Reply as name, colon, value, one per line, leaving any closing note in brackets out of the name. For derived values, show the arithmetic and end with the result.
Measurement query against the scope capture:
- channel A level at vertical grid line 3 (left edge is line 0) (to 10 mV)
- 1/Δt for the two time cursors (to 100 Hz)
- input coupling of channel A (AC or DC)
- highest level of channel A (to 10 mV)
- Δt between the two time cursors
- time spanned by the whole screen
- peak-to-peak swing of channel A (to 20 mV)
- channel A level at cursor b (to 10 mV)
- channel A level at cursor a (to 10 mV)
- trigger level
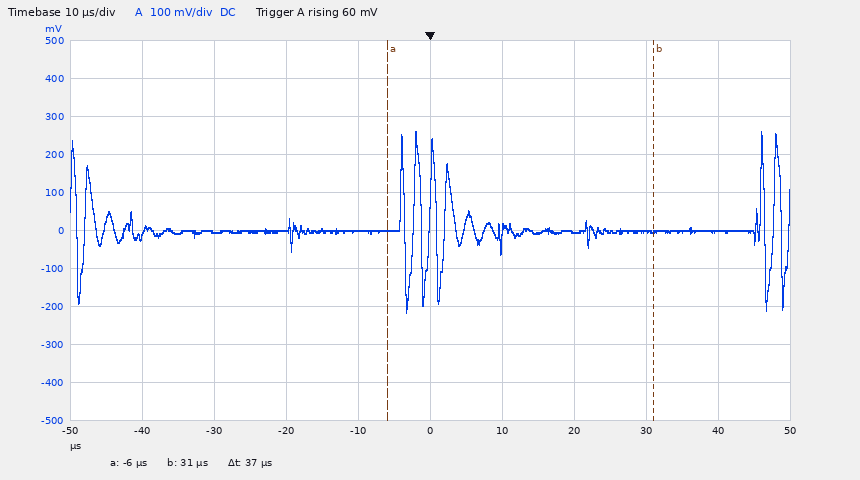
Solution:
channel A level at vertical grid line 3 (left edge is line 0): 0 mV
1/Δt for the two time cursors: 1 / 37 µs ≈ 27.0 kHz
input coupling of channel A: DC
highest level of channel A: 260 mV
Δt between the two time cursors: 37 µs
time spanned by the whole screen: 100 µs
peak-to-peak swing of channel A: 480 mV
channel A level at cursor b: 0 mV
channel A level at cursor a: 0 mV
trigger level: 60 mV
